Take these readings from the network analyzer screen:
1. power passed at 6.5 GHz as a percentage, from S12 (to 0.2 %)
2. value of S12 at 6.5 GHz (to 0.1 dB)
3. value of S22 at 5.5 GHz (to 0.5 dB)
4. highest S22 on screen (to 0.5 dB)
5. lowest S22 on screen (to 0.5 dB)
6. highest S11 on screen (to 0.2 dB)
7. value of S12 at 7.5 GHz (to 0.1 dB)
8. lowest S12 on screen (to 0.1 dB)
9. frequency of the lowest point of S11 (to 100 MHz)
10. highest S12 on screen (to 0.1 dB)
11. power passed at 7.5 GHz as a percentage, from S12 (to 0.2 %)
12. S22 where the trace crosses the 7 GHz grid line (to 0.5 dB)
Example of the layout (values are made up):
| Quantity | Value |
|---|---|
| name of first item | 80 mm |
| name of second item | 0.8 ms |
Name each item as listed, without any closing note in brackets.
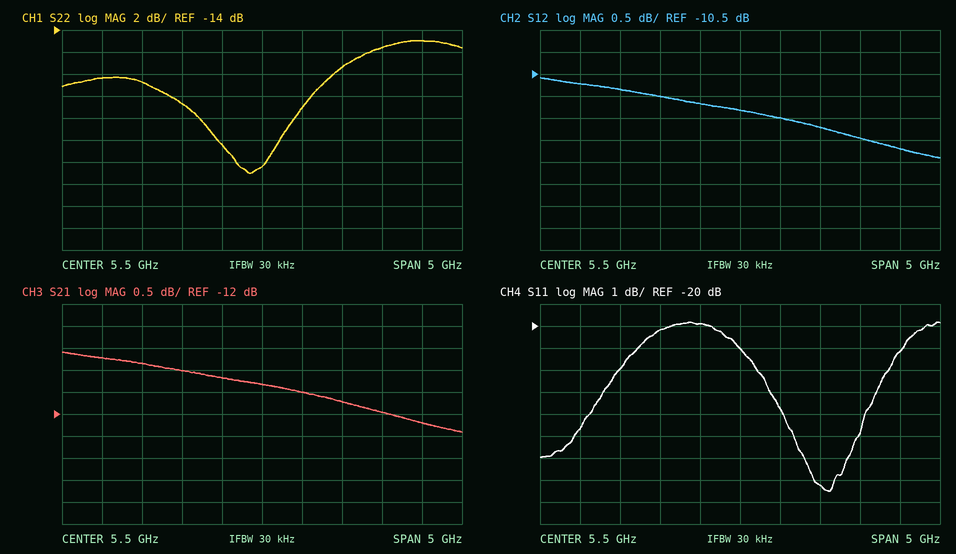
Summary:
| Quantity | Value |
|---|---|
| power passed at 6.5 GHz as a percentage, from S12 | 6.8 % |
| value of S12 at 6.5 GHz | -11.7 dB |
| value of S22 at 5.5 GHz | -26.5 dB |
| highest S22 on screen | -15.0 dB |
| lowest S22 on screen | -27.0 dB |
| highest S11 on screen | -19.8 dB |
| value of S12 at 7.5 GHz | -12.2 dB |
| lowest S12 on screen | -12.4 dB |
| frequency of the lowest point of S11 | 6.6 GHz |
| highest S12 on screen | -10.6 dB |
| power passed at 7.5 GHz as a percentage, from S12 | 6.0 % |
| S22 where the trace crosses the 7 GHz grid line | -15.5 dB |
